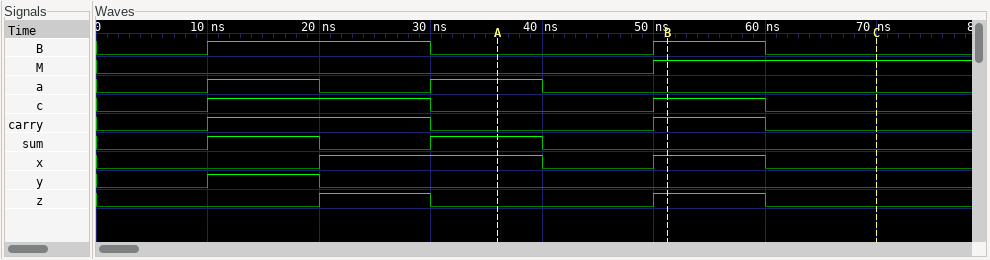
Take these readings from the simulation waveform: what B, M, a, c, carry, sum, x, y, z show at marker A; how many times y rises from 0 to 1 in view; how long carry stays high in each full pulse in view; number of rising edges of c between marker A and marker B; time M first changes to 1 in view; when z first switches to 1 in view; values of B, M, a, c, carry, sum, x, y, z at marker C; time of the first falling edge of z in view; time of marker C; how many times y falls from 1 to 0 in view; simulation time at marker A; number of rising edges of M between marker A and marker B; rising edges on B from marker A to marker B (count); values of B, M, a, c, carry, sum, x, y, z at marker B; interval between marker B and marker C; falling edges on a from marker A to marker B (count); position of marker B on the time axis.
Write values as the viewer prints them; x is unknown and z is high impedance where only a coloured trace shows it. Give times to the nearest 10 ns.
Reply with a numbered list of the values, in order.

1. B=0, M=0, a=1, c=0, carry=0, sum=1, x=1, y=0, z=0
2. 1
3. 20 ns, 10 ns
4. 1
5. 50 ns
6. 20 ns
7. B=0, M=1, a=0, c=0, carry=0, sum=0, x=0, y=0, z=0
8. 30 ns
9. 70 ns
10. 1
11. 40 ns
12. 1
13. 1
14. B=1, M=1, a=0, c=1, carry=1, sum=0, x=1, y=0, z=1
15. 20 ns
16. 1
17. 50 ns
